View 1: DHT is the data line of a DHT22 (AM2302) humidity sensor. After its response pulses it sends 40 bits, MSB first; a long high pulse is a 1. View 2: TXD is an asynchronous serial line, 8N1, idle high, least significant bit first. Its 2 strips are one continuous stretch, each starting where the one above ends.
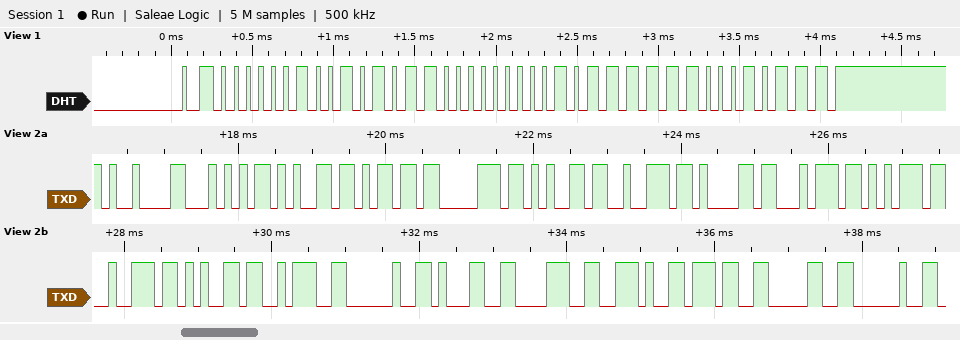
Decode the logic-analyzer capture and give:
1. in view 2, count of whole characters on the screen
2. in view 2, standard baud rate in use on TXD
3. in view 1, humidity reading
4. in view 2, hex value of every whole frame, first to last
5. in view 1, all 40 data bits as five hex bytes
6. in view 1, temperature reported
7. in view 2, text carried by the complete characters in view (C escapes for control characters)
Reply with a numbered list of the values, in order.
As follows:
1. 20
2. 9600 baud
3. 59.8 %
4. 09 54 65 6D 70 65 72 61 74 75 72 65 3A 20 31 38 2E 37 30 20
5. 02 56 00 BF 17
6. 19.1 °C
7. "\tTemperature: 18.70 "
